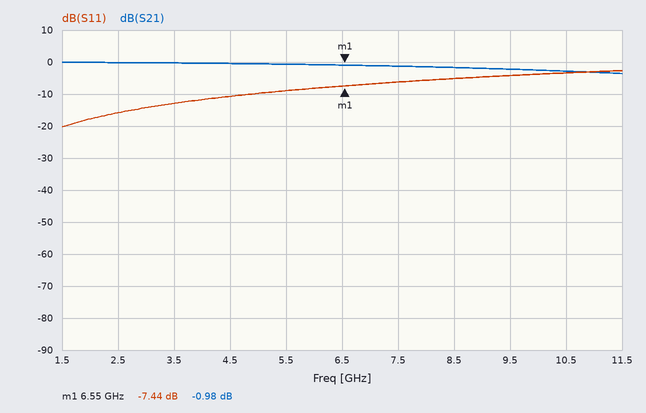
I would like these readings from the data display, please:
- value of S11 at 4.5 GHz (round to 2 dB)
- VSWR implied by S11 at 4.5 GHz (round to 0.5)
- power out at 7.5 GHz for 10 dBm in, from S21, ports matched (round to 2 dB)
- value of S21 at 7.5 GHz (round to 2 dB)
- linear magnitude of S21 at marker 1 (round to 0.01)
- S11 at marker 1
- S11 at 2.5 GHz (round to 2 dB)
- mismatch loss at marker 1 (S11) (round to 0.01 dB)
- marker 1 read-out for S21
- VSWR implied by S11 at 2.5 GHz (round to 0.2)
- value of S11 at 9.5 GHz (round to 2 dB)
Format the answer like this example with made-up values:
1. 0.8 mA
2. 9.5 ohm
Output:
1. -10 dB
2. 2.0
3. 8 dBm
4. -2 dB
5. 0.89
6. -7.44 dB
7. -16 dB
8. 0.86 dB
9. -0.98 dB
10. 1.4
11. -4 dB
